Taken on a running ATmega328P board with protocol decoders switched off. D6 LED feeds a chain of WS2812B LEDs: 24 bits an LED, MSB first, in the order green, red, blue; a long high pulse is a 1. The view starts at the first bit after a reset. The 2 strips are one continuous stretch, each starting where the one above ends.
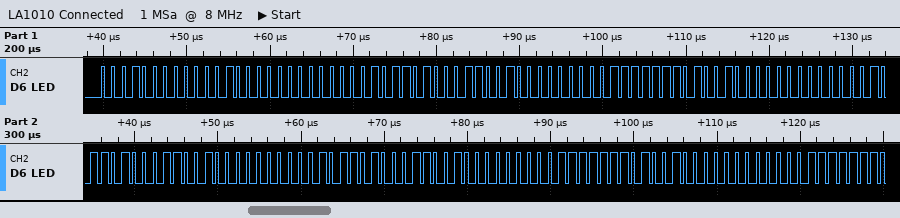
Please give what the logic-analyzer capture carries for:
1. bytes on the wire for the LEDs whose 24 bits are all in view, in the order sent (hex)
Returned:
10 08 00 2D 19 00 7F 48 00 2D 19 00 2D 19 00 7F 48 00
